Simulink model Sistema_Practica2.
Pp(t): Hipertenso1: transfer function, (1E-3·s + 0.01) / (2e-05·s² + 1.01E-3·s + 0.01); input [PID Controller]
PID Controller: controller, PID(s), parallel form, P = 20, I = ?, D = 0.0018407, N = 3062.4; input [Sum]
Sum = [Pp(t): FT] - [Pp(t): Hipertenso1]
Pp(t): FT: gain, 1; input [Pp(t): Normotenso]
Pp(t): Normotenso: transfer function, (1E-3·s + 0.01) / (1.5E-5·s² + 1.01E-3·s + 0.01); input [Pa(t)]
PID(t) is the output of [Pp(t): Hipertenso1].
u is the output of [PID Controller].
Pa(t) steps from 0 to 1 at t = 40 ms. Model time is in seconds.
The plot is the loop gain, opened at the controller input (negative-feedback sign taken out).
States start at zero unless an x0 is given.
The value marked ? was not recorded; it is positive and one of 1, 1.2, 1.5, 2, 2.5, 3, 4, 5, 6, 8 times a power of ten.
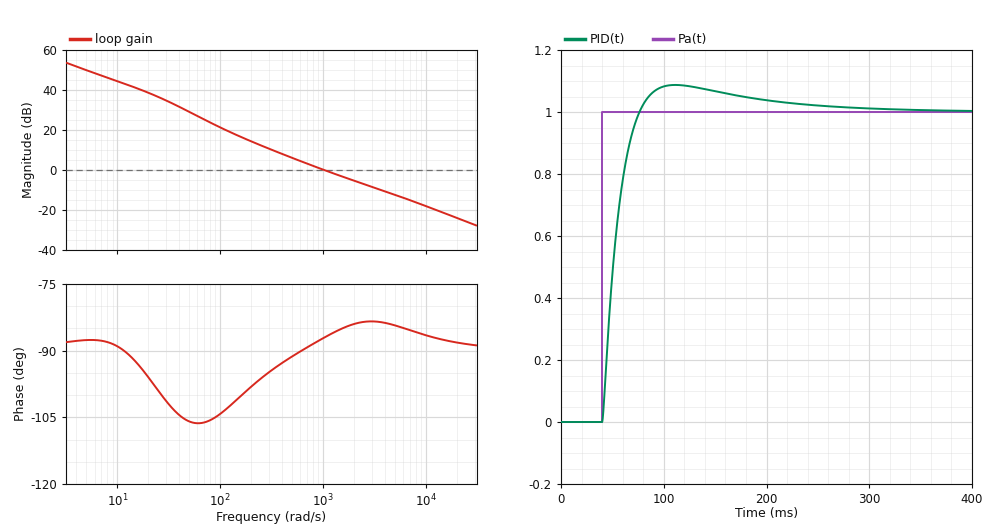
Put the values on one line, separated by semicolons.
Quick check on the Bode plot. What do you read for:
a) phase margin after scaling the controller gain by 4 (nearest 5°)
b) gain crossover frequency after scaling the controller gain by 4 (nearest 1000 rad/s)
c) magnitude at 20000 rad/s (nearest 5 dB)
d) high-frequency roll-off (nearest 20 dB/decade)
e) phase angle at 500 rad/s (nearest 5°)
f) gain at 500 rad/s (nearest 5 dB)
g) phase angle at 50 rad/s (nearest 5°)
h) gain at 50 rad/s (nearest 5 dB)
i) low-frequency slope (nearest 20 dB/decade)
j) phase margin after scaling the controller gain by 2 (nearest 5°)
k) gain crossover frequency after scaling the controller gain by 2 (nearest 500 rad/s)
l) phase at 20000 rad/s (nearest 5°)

95°; 5000 rad/s; -25 dB; -20 dB/decade; -90°; 5 dB; -105°; 30 dB; -20 dB/decade; 95°; 2000 rad/s; -90°
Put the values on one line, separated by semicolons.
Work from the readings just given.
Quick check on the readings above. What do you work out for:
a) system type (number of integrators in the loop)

1
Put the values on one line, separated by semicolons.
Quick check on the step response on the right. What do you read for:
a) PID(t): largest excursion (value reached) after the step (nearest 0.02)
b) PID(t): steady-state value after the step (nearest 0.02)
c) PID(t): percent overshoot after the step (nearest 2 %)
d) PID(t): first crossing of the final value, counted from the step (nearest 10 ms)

1.08; 1.00; 8 %; 40 ms
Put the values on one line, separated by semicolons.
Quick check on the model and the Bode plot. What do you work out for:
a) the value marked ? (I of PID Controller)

1500
